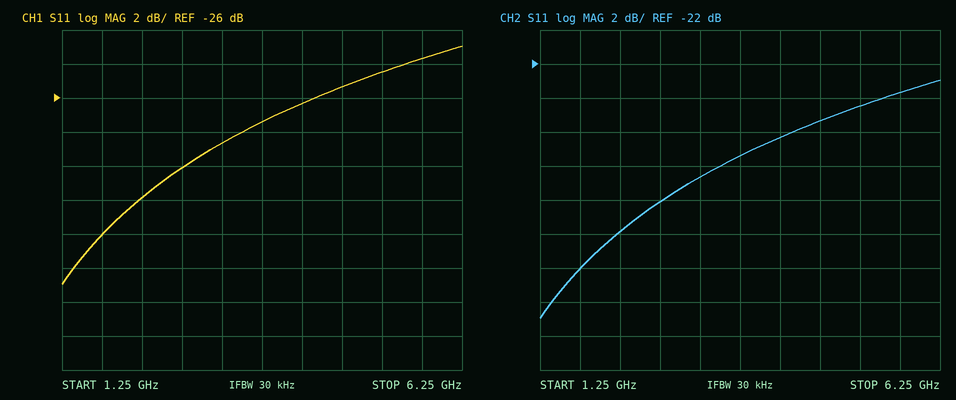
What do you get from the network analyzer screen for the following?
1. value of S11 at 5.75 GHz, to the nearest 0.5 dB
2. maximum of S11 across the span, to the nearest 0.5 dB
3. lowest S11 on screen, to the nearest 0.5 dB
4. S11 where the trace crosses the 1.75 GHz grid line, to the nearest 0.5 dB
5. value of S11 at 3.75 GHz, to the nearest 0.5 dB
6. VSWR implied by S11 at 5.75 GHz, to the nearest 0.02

-23.5 dB
-23.0 dB
-37.0 dB
-34.0 dB
-27.5 dB
1.14
